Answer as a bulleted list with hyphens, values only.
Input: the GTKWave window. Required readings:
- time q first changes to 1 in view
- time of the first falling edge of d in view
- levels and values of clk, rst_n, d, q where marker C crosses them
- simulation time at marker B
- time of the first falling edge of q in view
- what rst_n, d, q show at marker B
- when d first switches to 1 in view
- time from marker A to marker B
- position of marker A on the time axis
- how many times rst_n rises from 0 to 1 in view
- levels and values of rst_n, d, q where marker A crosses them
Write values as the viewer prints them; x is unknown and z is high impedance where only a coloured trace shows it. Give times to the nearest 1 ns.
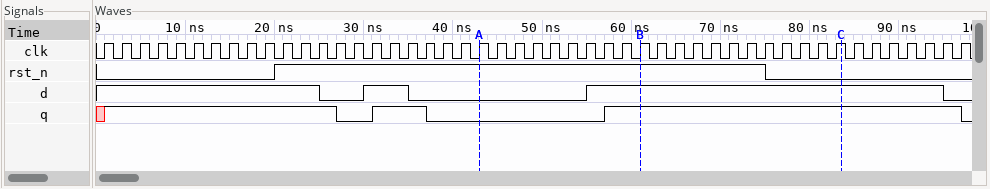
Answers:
- 1 ns
- 25 ns
- clk=1, rst_n=0, d=1, q=1
- 61 ns
- 27 ns
- rst_n=1, d=1, q=1
- 30 ns
- 18 ns
- 43 ns
- 1
- rst_n=1, d=0, q=0
